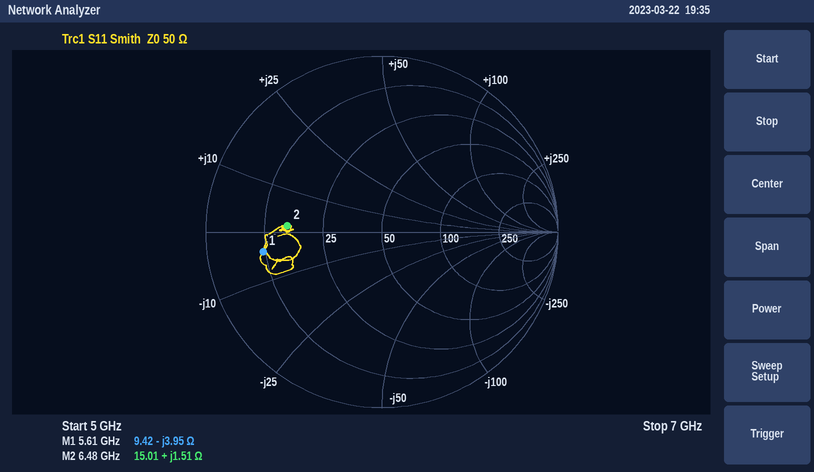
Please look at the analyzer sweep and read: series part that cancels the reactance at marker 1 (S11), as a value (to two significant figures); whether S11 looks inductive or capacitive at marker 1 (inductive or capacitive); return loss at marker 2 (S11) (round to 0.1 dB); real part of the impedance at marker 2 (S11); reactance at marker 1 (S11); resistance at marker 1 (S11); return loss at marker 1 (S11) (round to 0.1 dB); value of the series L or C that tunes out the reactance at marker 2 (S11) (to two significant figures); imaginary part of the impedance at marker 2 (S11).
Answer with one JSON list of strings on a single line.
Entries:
["110 pH", "capacitive", "5.4 dB", "15.01 Ω", "-3.95 Ω", "9.42 Ω", "3.3 dB", "16 pF", "+1.51 Ω"]
